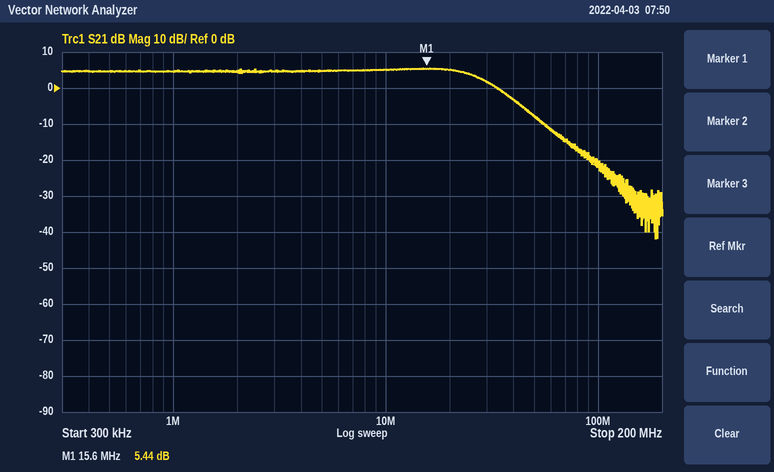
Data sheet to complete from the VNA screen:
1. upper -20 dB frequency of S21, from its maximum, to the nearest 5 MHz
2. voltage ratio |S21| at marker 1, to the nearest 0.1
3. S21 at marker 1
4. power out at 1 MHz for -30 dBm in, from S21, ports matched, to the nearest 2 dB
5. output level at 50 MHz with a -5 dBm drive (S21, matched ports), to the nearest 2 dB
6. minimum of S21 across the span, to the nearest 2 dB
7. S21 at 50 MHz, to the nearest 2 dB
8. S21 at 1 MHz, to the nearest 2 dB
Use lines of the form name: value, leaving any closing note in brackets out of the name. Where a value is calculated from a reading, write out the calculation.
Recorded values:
upper -20 dB frequency of S21, from its maximum, to the nearest 5 MHz: 70 MHz
voltage ratio |S21| at marker 1, to the nearest 0.1: 10^(5.44/20) ≈ 1.9
S21 at marker 1: 5.44 dB
power out at 1 MHz for -30 dBm in, from S21, ports matched, to the nearest 2 dB: -30 dBm + (4 dB) = -26 dBm
output level at 50 MHz with a -5 dBm drive (S21, matched ports), to the nearest 2 dB: -5 dBm + (-8 dB) = -12 dBm
minimum of S21 across the span, to the nearest 2 dB: -42 dB
S21 at 50 MHz, to the nearest 2 dB: -8 dB
S21 at 1 MHz, to the nearest 2 dB: 4 dB
